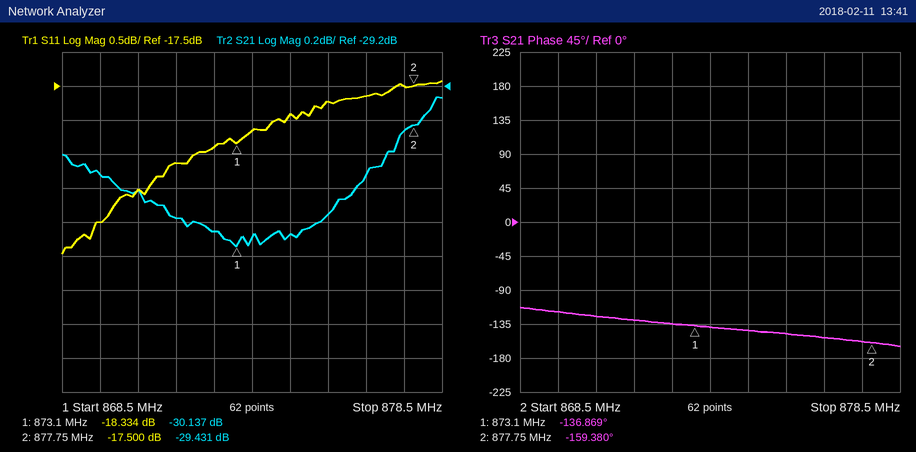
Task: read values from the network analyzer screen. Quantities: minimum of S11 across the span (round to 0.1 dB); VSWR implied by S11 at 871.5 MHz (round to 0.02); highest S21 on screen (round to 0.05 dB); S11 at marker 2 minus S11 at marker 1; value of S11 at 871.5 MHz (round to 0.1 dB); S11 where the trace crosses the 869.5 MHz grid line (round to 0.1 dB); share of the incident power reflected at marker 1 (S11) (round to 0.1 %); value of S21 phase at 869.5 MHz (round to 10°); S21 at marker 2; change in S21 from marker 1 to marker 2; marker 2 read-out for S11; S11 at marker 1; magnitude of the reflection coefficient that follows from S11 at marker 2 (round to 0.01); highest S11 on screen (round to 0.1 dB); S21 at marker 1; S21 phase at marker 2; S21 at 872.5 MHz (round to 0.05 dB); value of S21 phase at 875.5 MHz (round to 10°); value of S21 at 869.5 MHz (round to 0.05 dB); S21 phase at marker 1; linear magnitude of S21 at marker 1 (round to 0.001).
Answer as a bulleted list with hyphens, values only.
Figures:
- -20.0 dB
- 1.26
- -29.25 dB
- 0.834 dB
- -18.6 dB
- -19.5 dB
- 1.5 %
- -120°
- -29.431 dB
- 0.706 dB
- -17.500 dB
- -18.334 dB
- 0.13
- -17.4 dB
- -30.137 dB
- -159.380°
- -30.05 dB
- -150°
- -29.70 dB
- -136.869°
- 0.031
